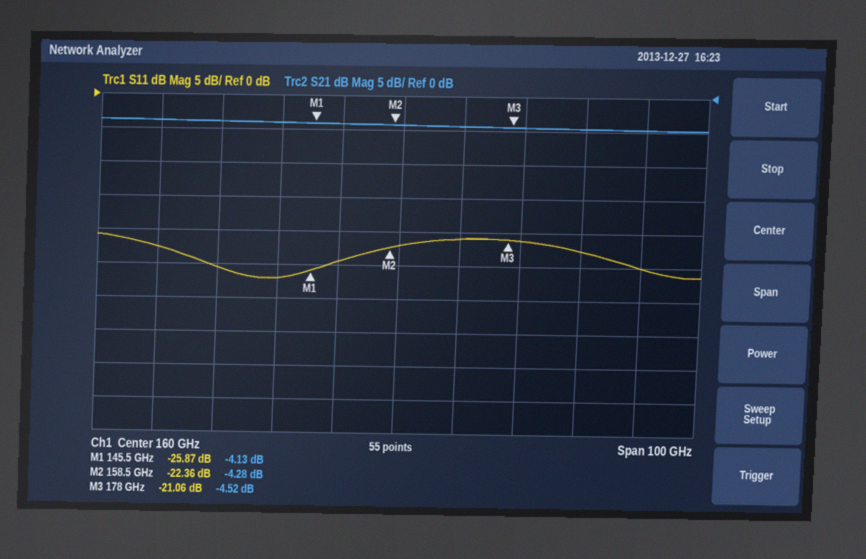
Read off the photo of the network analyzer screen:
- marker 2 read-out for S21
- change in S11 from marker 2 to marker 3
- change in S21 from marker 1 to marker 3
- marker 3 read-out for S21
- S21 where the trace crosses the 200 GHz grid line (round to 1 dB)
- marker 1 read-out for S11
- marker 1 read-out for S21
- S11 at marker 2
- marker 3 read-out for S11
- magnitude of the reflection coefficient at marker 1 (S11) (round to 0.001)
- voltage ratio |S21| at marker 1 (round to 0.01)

-4.28 dB
1.30 dB
-0.39 dB
-4.52 dB
-5 dB
-25.87 dB
-4.13 dB
-22.36 dB
-21.06 dB
0.051
0.62
